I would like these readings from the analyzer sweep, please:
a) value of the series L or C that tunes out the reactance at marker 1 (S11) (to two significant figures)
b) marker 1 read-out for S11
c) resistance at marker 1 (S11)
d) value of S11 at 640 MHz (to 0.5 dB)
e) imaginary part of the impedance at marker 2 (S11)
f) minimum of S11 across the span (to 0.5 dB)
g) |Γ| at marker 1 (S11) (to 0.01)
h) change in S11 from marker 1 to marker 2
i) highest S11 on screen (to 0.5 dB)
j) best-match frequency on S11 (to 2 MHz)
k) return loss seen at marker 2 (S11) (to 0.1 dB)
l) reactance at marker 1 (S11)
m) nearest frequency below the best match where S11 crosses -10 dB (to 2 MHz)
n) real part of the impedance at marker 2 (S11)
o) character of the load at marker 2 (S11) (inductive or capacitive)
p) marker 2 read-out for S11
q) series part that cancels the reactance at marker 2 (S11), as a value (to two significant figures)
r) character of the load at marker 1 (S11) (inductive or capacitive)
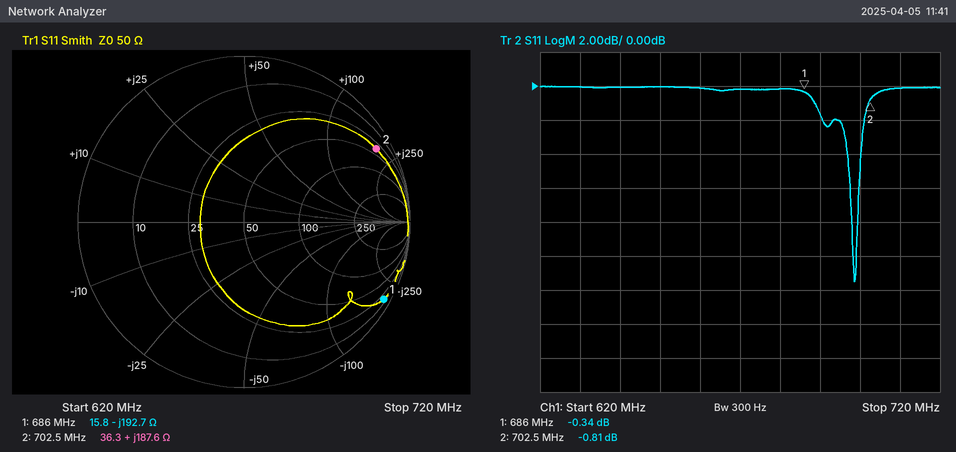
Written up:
45 nH
-0.34 dB
15.8 Ω
0.0 dB
+187.6 Ω
-11.5 dB
0.96
-0.47 dB
0.0 dB
698 MHz
0.8 dB
-192.7 Ω
698 MHz
36.3 Ω
inductive
-0.81 dB
1.2 pF
capacitive
